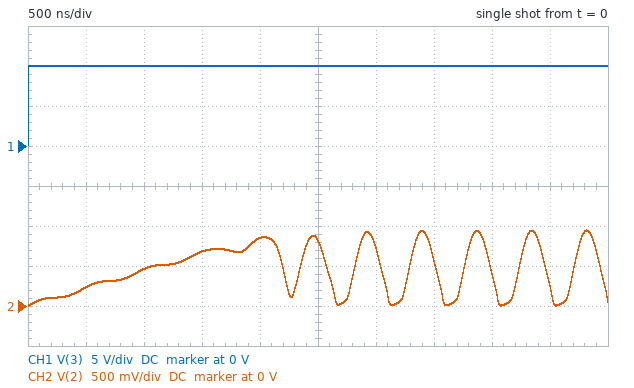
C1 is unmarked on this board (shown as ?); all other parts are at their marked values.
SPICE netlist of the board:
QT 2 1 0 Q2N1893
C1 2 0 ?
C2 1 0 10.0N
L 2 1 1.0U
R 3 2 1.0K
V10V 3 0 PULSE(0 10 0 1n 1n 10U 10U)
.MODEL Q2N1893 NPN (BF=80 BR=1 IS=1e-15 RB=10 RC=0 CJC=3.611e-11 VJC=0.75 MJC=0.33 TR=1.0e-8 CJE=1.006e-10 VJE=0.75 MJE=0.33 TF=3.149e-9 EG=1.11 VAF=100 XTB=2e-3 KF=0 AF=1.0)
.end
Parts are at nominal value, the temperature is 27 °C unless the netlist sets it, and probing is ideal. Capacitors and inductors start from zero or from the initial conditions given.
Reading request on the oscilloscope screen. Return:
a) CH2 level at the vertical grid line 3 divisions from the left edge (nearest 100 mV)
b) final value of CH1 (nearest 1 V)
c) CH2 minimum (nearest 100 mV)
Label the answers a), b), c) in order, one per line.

a) 700 mV
b) 10 V
c) 0 V
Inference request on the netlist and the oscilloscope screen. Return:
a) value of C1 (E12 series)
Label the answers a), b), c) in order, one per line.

a) 12 nF
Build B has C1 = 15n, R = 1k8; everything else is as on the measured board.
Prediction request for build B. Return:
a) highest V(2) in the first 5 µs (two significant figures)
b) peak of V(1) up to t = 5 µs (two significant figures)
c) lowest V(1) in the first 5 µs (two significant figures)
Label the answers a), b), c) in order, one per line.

a) 800 mV
b) 880 mV
c) -150 mV
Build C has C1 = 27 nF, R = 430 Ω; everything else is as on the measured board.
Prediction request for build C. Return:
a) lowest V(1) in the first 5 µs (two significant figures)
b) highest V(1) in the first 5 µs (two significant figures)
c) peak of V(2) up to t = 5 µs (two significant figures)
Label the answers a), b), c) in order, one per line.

a) -420 mV
b) 1.1 V
c) 800 mV
